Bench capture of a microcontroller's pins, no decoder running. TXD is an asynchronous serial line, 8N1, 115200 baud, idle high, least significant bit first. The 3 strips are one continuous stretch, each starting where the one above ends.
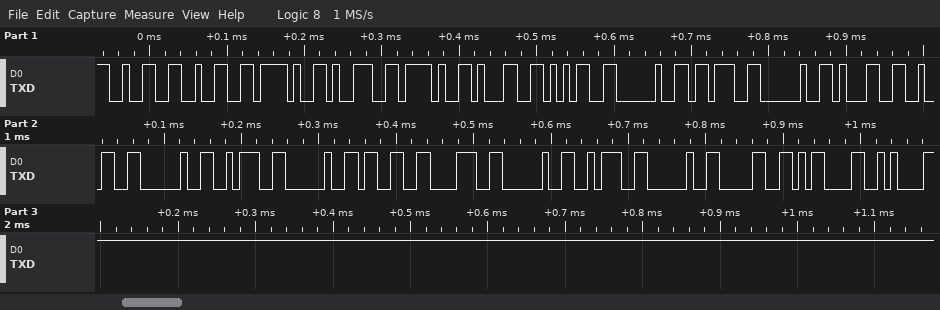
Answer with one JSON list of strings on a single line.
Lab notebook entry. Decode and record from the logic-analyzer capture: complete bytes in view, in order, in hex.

["0x32 0x32 0x2F 0x39 0x2F 0x31 0x35 0x20 0x3B 0x20 0x31 0x32 0x20 0x3A 0x20 0x33 0x38 0x20 0x3A 0x20 0x30 0x0D 0x0A"]
